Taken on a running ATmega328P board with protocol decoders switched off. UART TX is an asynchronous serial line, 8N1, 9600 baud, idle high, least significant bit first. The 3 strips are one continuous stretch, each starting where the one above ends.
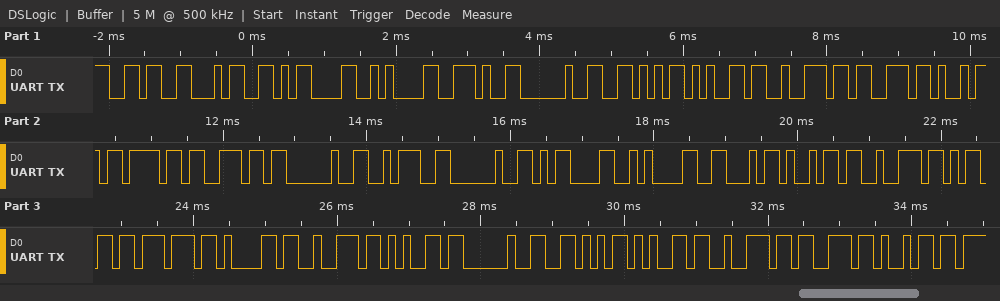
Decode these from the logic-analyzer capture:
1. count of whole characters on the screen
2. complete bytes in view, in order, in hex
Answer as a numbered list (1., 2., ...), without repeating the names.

1. 32
2. 36 34 0D 0A 2E 20 56 65 72 73 69 6F 6E 20 3A 20 0D 0A 46 69 72 6D 77 61 72 65 20 56 65 72 73 69
